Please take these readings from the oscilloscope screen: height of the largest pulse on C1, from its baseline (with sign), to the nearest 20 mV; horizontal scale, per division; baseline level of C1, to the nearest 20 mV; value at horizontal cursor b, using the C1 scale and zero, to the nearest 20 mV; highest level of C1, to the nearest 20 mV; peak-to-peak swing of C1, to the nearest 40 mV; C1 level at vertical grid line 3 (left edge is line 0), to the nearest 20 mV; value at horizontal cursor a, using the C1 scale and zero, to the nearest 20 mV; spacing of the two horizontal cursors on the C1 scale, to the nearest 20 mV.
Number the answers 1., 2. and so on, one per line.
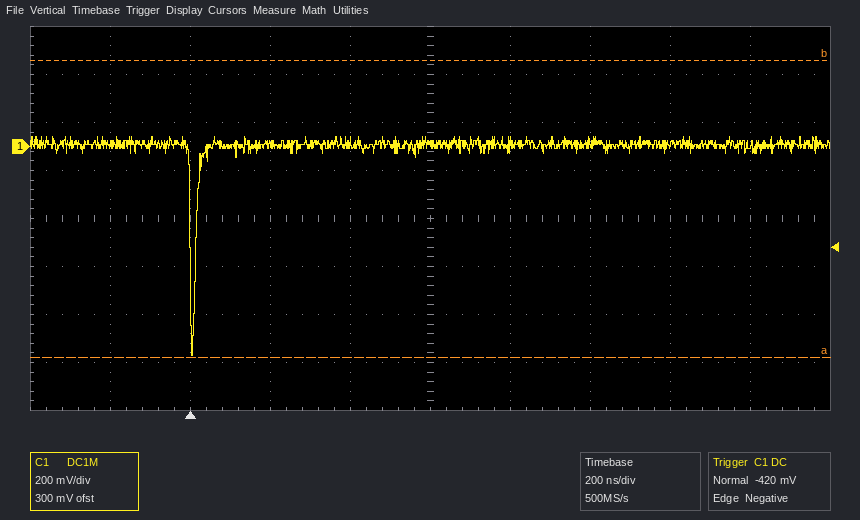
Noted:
1. -880 mV
2. 200 ns
3. 0 mV
4. 360 mV
5. 40 mV
6. 920 mV
7. 0 mV
8. -880 mV
9. 1.24 V
